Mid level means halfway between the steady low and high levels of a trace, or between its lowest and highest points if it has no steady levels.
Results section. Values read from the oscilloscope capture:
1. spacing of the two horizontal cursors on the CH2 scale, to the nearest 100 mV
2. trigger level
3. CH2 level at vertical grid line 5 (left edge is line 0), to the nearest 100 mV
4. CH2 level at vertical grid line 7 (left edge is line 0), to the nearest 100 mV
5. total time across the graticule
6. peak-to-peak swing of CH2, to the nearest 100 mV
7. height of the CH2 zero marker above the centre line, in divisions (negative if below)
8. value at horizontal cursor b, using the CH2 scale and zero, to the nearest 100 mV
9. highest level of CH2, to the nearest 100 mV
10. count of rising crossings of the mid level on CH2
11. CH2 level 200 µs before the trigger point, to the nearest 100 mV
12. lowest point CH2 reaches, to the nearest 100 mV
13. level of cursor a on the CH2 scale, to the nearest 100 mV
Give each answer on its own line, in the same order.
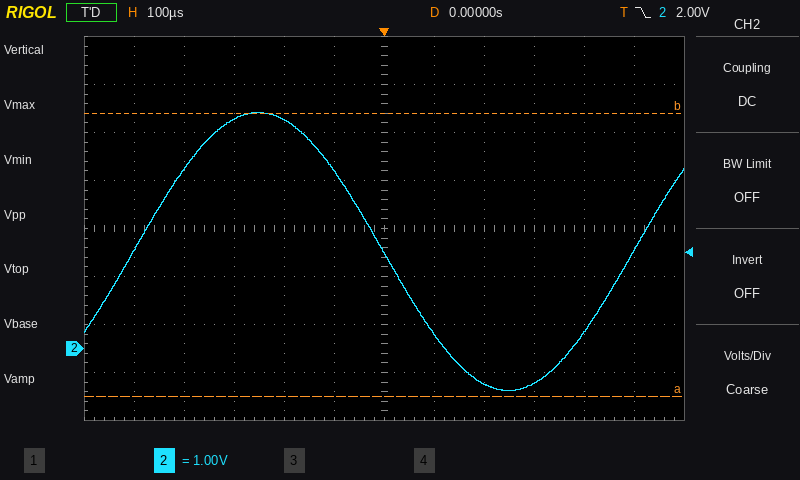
5.9 V
2.00 V
3.7 V
300 mV
1.2 ms
5.8 V
-2.5 div
4.9 V
4.9 V
2
4.8 V
-900 mV
-1.0 V
